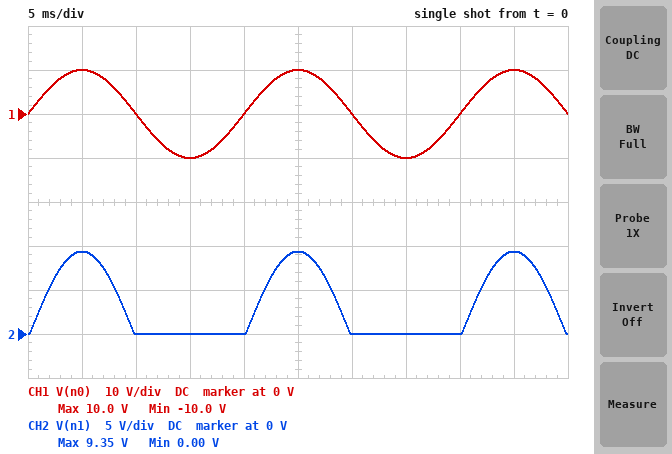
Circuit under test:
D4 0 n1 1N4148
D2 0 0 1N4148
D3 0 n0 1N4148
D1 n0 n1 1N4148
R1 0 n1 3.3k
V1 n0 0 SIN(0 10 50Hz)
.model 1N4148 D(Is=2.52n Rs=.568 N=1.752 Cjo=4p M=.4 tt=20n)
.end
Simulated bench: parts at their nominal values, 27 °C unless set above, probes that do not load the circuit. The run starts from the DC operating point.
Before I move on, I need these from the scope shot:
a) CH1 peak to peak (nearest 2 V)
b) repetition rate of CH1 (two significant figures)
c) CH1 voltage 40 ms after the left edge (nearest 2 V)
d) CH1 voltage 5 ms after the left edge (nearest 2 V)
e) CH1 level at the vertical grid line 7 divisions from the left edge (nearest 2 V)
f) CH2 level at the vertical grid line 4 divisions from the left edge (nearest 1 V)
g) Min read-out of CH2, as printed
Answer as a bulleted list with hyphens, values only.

- 20 V
- 50 Hz
- 0 V
- 10 V
- -10 V
- 0 V
- 0.00 V
